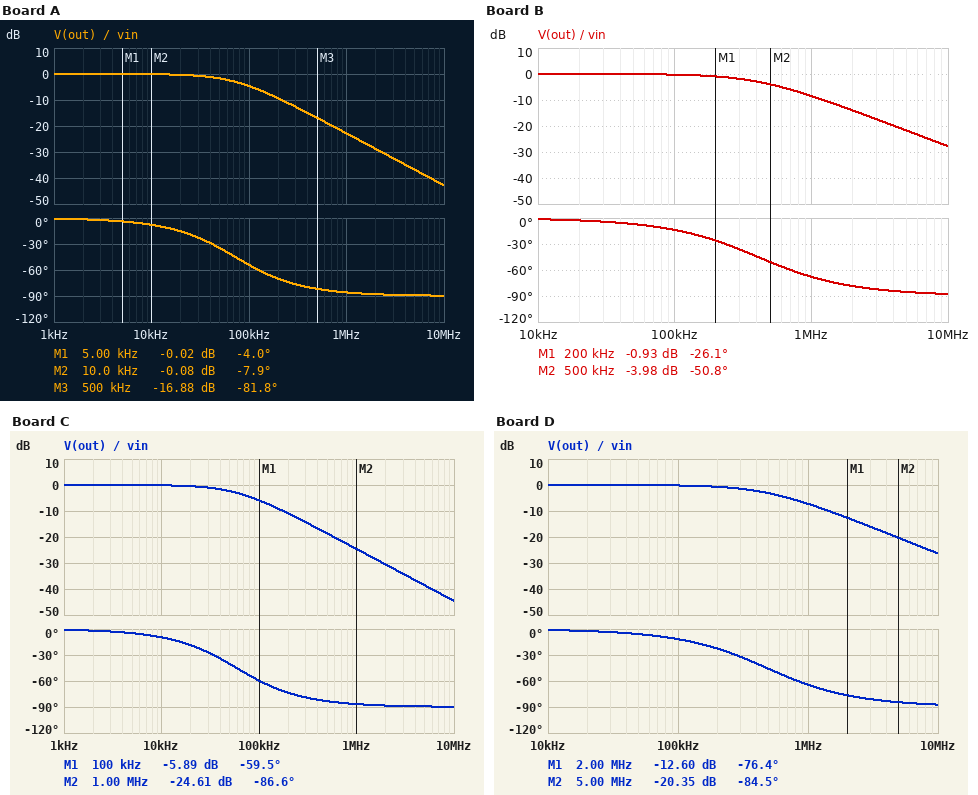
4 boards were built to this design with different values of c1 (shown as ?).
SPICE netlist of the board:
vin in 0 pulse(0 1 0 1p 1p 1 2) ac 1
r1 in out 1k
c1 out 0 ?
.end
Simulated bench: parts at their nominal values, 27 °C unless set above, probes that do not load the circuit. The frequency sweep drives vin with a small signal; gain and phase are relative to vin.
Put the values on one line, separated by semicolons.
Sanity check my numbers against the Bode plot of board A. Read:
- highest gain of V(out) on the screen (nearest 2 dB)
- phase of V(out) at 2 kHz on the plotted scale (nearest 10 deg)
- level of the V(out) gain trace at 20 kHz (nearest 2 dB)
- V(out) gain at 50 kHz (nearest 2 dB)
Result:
0 dB; 0 deg; 0 dB; -2 dB
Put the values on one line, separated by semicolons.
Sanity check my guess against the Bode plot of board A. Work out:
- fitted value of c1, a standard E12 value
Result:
2.2 nF
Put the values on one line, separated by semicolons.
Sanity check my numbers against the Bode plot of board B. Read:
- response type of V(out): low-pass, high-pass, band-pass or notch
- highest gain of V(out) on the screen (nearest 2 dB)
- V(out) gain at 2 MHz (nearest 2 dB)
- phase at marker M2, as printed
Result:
low-pass; 0 dB; -14 dB; -50.8 deg
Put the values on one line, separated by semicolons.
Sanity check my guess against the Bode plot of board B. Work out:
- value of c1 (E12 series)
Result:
390 pF
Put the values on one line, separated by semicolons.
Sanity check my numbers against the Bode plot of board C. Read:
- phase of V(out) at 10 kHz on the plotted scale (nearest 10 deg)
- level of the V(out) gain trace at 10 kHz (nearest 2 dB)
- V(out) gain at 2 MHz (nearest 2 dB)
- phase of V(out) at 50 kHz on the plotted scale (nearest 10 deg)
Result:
-10 deg; 0 dB; -30 dB; -40 deg
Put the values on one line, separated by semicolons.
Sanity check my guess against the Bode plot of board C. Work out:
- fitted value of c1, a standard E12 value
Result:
2.7 nF
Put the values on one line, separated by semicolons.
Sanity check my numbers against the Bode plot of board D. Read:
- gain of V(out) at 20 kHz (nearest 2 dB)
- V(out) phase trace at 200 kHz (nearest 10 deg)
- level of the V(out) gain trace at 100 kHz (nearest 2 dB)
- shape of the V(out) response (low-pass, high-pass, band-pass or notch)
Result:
0 dB; -20 deg; 0 dB; low-pass
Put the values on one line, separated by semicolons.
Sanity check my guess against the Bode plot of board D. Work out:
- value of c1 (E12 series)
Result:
330 pF
